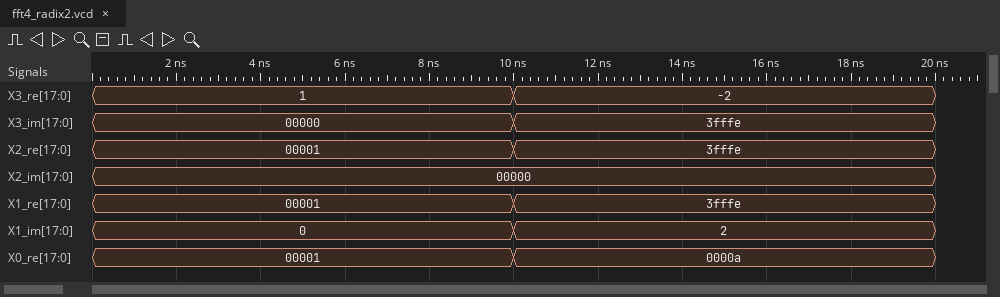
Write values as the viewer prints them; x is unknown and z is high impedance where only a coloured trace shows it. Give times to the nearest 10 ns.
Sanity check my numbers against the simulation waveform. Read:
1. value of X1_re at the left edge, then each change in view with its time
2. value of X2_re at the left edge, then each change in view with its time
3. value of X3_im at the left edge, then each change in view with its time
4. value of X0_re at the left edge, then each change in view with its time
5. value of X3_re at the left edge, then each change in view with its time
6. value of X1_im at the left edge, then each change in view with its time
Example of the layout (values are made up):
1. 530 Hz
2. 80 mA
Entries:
1. 00001, 3fffe at 10 ns
2. 00001, 3fffe at 10 ns
3. 00000, 3fffe at 10 ns
4. 00001, 0000a at 10 ns
5. 1, -2 at 10 ns
6. 0, 2 at 10 ns
